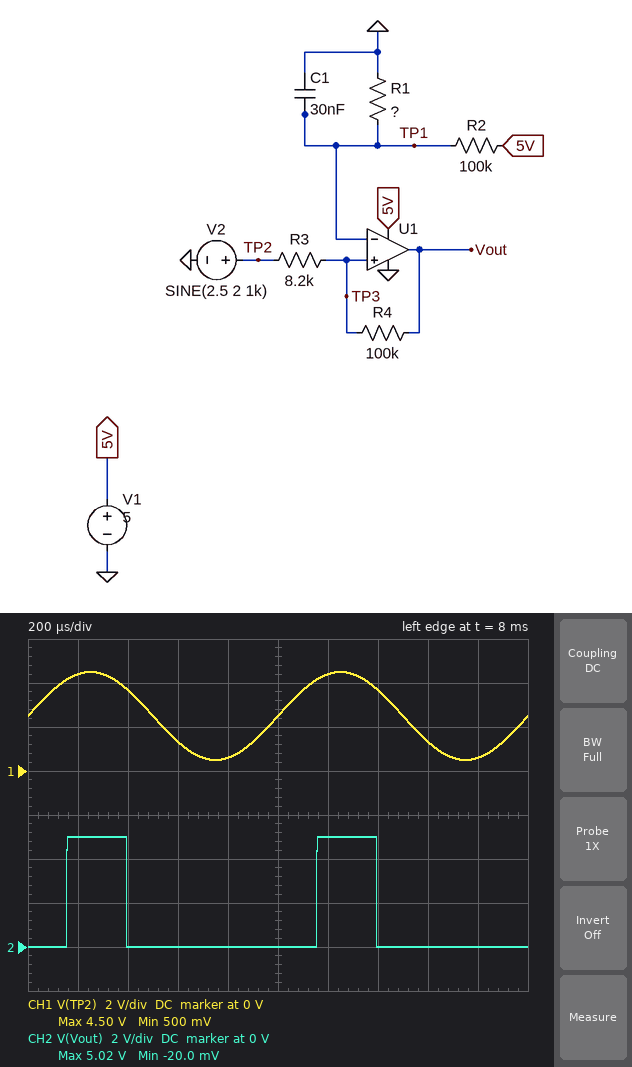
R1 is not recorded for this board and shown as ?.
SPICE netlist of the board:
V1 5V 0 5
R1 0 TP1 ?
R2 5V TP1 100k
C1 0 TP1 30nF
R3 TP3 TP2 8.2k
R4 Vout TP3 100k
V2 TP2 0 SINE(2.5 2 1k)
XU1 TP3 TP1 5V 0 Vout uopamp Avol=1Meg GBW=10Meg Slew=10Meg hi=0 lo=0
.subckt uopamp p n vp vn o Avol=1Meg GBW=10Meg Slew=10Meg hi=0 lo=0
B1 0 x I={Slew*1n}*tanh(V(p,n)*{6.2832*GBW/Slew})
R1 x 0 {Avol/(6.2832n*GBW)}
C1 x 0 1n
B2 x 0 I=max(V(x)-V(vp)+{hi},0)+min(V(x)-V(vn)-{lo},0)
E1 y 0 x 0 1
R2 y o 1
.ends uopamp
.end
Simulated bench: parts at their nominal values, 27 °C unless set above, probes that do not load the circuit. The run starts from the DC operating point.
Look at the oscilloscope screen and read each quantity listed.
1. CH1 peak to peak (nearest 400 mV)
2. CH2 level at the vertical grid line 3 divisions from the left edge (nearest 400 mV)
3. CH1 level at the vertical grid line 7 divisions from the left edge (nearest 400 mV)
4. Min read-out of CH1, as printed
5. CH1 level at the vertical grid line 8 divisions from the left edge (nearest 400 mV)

4.0 V
0 V
3.6 V
500 mV
1.2 V
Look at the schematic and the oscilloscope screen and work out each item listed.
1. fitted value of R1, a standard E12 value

330 kΩ
